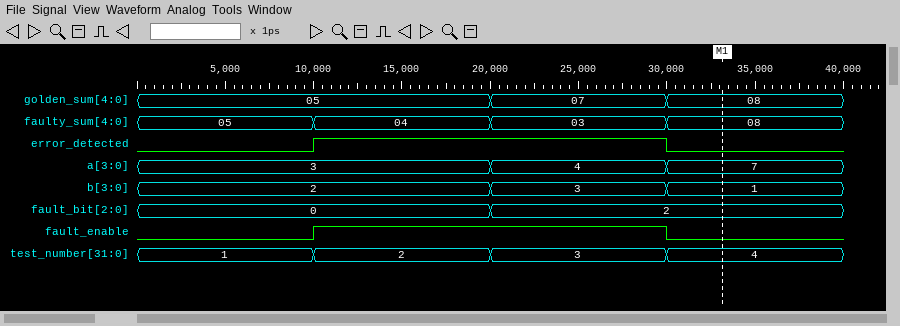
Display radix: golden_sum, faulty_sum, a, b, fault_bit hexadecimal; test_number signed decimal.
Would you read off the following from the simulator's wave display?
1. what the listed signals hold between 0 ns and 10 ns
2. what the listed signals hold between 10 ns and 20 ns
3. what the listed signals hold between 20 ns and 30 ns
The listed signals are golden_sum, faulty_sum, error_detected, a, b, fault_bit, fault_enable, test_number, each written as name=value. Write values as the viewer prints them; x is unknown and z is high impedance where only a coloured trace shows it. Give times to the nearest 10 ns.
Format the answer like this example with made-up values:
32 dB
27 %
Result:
golden_sum=05, faulty_sum=05, error_detected=0, a=3, b=2, fault_bit=0, fault_enable=0, test_number=1
golden_sum=05, faulty_sum=04, error_detected=1, a=3, b=2, fault_bit=0, fault_enable=1, test_number=2
golden_sum=07, faulty_sum=03, error_detected=1, a=4, b=3, fault_bit=2, fault_enable=1, test_number=3
